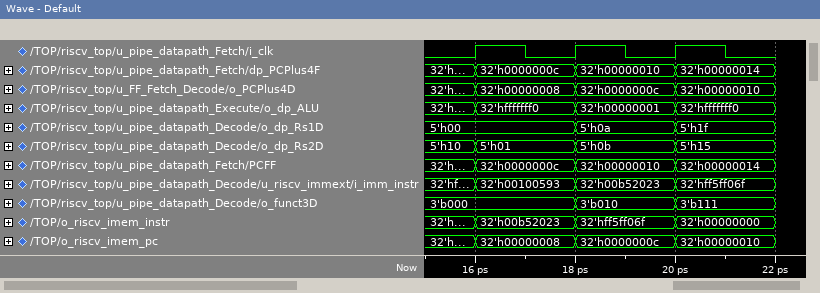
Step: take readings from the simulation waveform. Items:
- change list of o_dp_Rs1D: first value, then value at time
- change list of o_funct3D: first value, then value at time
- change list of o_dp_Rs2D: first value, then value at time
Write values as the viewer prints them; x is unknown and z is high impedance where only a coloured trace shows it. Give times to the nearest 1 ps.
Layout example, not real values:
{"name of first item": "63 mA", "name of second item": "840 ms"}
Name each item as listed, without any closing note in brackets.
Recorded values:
{"change list of o_dp_Rs1D: first value, then value at time": "5'h00, 5'h0a at 18 ps, 5'h1f at 20 ps", "change list of o_funct3D: first value, then value at time": "3'b000, 3'b010 at 18 ps, 3'b111 at 20 ps", "change list of o_dp_Rs2D: first value, then value at time": "5'h10, 5'h01 at 16 ps, 5'h0b at 18 ps, 5'h15 at 20 ps"}
